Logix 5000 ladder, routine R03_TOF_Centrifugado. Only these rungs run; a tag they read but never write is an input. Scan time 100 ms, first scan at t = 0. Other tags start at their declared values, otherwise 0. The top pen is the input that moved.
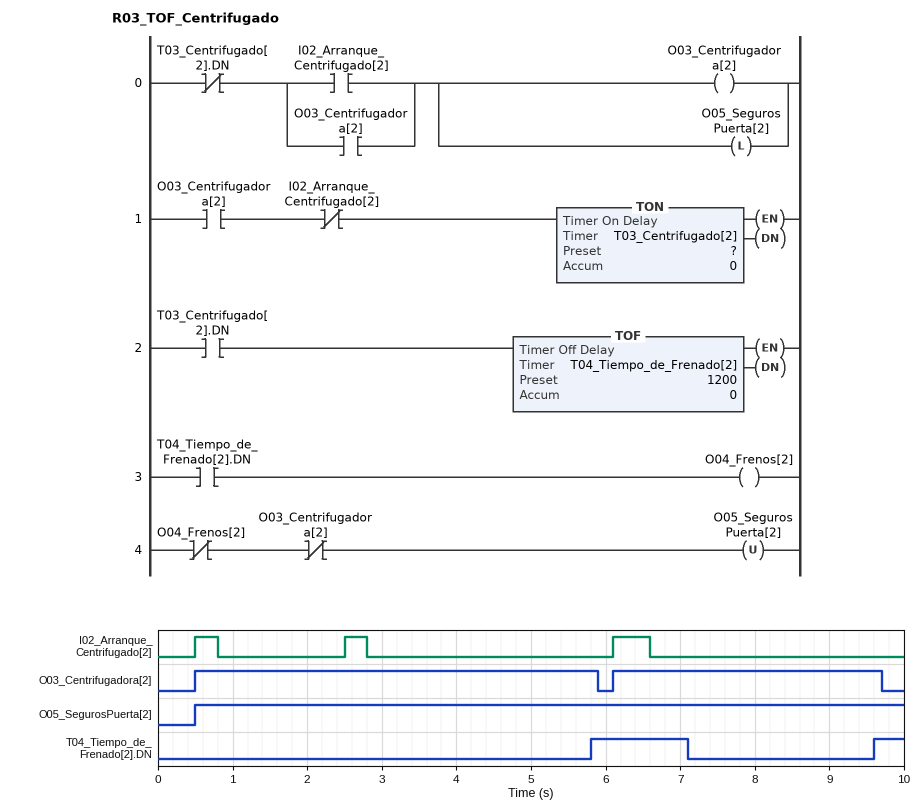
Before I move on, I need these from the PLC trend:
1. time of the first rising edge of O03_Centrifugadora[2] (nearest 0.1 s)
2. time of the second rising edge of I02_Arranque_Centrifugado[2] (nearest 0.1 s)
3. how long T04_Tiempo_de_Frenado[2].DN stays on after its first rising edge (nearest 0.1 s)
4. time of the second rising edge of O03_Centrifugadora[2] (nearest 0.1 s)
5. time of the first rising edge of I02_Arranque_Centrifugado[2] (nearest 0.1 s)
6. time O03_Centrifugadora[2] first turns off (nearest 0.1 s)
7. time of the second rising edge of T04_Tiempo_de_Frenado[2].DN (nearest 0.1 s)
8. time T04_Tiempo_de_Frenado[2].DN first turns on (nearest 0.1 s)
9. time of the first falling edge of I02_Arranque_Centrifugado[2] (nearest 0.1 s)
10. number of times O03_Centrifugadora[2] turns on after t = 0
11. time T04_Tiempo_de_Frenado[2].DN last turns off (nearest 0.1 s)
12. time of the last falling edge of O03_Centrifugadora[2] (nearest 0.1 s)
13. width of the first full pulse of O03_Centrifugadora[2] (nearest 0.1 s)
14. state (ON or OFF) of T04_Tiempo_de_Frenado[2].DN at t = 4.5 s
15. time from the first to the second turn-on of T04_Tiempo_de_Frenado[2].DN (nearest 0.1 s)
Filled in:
0.5 s
2.5 s
1.3 s
6.1 s
0.5 s
5.9 s
9.6 s
5.8 s
0.8 s
2
7.1 s
9.7 s
5.4 s
OFF
3.8 s
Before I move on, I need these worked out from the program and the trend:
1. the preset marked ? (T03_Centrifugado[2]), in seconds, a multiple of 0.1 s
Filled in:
3.0 s
